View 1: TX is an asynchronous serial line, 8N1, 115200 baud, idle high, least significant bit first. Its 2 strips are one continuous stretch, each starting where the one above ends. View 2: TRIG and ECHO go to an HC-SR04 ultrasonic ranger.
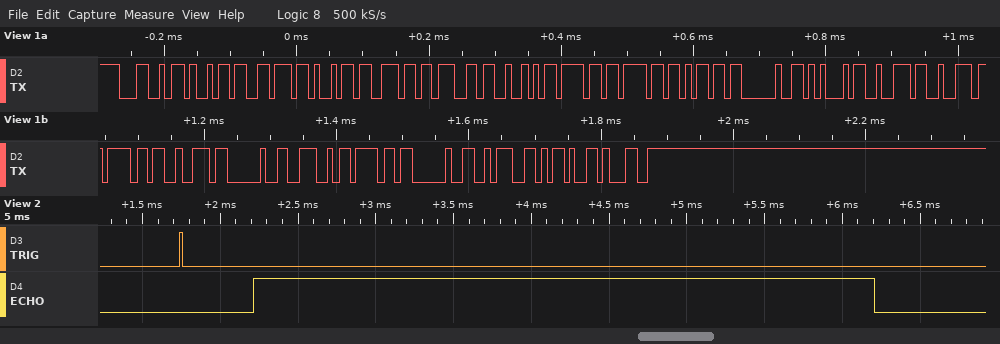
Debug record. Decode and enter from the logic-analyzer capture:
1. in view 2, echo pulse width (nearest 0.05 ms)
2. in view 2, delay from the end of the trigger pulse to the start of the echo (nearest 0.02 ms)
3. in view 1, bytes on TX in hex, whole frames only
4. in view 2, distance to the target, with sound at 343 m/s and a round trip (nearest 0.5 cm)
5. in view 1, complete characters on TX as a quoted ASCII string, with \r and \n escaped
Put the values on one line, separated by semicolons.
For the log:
4.00 ms; 0.46 ms; 4C 69 76 69 6E 67 52 6F 6F 6D 20 45 72 72 6F 72 20 4E 6F 20 3A 2D 31; 68.5 cm; "LivingRoom Error No :-1"
